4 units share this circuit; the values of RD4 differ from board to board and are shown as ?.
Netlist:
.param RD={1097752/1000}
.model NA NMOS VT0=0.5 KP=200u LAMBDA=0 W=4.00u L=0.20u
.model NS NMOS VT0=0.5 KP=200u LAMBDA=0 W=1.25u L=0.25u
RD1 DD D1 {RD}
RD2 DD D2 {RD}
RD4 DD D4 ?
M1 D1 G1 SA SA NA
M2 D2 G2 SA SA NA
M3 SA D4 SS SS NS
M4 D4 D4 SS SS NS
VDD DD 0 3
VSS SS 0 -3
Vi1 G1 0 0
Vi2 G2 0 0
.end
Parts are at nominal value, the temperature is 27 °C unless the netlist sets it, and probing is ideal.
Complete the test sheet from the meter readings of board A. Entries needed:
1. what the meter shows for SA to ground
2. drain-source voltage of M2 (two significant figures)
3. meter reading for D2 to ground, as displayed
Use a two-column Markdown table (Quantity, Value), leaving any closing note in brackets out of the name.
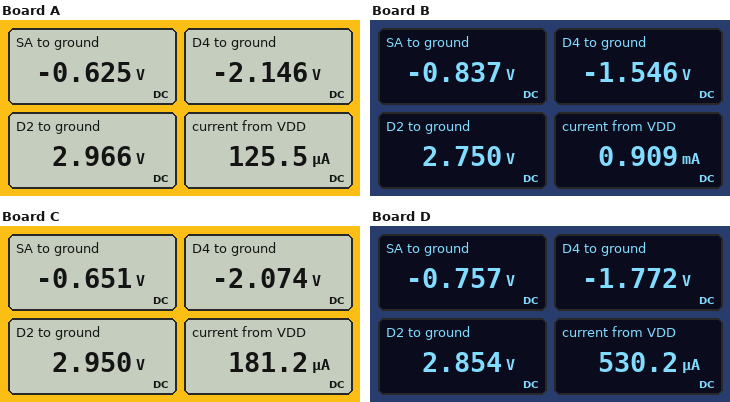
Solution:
| Quantity | Value |
|---|---|
| what the meter shows for SA to ground | -0.625 V |
| drain-source voltage of M2 | 3.6 V |
| meter reading for D2 to ground, as displayed | 2.966 V |
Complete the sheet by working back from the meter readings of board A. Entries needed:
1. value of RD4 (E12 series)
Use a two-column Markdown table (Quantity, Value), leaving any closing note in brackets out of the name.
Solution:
| Quantity | Value |
|---|---|
| value of RD4 | 82 kΩ |
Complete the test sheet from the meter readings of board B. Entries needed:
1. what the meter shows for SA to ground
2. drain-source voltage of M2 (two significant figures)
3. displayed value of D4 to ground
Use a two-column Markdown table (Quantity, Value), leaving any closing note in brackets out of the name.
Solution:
| Quantity | Value |
|---|---|
| what the meter shows for SA to ground | -0.837 V |
| drain-source voltage of M2 | 3.6 V |
| displayed value of D4 to ground | -1.546 V |
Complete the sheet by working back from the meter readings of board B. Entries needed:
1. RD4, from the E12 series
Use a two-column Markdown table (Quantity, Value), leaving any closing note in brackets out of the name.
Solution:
| Quantity | Value |
|---|---|
| RD4, from the E12 series | 10 kΩ |
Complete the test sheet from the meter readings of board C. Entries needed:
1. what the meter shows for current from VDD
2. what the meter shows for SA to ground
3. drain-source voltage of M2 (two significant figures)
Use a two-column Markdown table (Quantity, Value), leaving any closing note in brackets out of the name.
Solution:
| Quantity | Value |
|---|---|
| what the meter shows for current from VDD | 181.2 µA |
| what the meter shows for SA to ground | -0.651 V |
| drain-source voltage of M2 | 3.6 V |
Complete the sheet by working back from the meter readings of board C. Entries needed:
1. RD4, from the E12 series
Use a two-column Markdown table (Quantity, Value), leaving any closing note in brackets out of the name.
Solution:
| Quantity | Value |
|---|---|
| RD4, from the E12 series | 56 kΩ |
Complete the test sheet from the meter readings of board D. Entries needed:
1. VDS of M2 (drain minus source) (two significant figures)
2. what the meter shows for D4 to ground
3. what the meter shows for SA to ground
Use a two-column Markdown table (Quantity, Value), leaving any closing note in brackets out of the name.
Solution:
| Quantity | Value |
|---|---|
| VDS of M2 (drain minus source) | 3.6 V |
| what the meter shows for D4 to ground | -1.772 V |
| what the meter shows for SA to ground | -0.757 V |
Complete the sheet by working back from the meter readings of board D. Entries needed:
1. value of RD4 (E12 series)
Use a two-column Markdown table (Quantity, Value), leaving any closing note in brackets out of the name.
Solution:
| Quantity | Value |
|---|---|
| value of RD4 | 18 kΩ |
